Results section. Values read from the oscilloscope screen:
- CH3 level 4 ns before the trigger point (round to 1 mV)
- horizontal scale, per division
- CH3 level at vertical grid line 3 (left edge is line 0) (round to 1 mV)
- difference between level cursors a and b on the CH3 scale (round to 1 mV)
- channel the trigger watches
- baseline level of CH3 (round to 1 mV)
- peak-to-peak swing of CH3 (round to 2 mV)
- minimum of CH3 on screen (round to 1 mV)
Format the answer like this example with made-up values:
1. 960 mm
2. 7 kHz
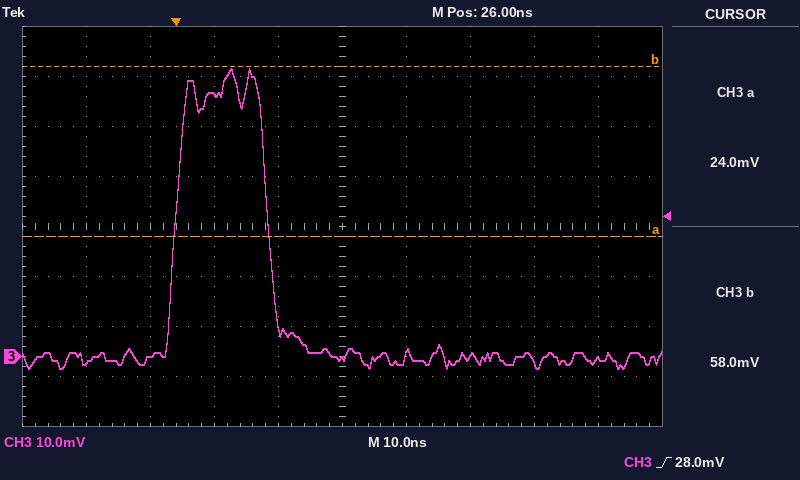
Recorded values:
1. 0 mV
2. 10 ns
3. 52 mV
4. 34 mV
5. CH3
6. 0 mV
7. 60 mV
8. -2 mV
